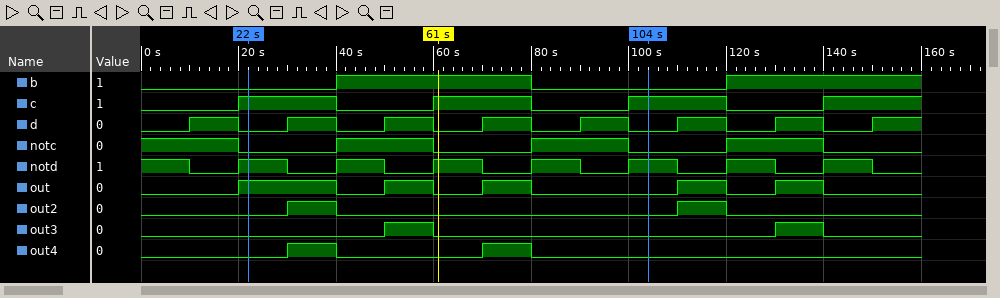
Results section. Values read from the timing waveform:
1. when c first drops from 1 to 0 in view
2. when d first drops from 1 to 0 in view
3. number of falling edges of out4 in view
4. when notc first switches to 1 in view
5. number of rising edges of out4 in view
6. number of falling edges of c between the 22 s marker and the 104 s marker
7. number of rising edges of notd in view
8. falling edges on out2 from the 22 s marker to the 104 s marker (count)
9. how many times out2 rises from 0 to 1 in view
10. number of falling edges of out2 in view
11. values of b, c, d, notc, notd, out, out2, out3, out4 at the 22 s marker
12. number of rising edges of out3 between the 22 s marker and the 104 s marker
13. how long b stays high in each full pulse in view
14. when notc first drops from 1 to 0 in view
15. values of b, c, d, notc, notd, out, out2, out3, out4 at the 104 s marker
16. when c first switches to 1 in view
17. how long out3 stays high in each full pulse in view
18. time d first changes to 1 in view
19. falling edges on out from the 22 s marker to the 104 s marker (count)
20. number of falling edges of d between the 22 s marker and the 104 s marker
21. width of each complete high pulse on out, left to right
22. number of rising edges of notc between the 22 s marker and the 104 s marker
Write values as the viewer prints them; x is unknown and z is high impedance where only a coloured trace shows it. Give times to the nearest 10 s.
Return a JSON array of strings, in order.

["40 s", "20 s", "2", "40 s", "2", "2", "7", "1", "2", "2", "b=0, c=1, d=0, notc=0, notd=1, out=1, out2=0, out3=0, out4=0", "1", "40 s", "20 s", "b=0, c=1, d=0, notc=0, notd=1, out=0, out2=0, out3=0, out4=0", "20 s", "10 s, 10 s", "10 s", "3", "4", "20 s, 10 s, 10 s, 10 s, 10 s", "2"]
